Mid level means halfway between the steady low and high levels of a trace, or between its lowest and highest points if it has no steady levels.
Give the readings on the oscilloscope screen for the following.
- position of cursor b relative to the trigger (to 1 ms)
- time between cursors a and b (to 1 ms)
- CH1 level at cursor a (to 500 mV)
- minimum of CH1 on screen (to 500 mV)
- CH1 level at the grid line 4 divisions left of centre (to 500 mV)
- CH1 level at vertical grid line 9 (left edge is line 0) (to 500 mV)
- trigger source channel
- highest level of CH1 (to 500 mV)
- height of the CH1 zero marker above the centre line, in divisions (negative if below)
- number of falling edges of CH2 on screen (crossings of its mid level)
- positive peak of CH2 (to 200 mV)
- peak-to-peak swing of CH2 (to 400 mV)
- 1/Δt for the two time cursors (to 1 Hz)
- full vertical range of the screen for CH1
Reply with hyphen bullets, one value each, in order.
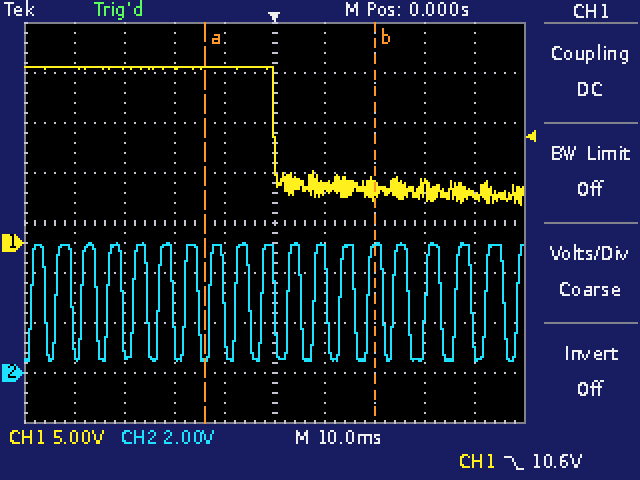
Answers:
- +20 ms
- 34 ms
- 17.5 V
- 4.0 V
- 17.5 V
- 5.0 V
- CH1
- 17.5 V
- -0.4 div
- 18
- 5.2 V
- 4.8 V
- 29 Hz
- 40 V
